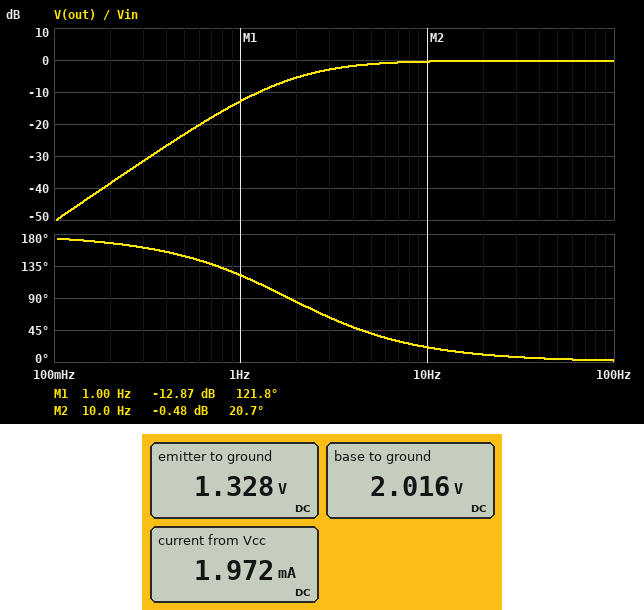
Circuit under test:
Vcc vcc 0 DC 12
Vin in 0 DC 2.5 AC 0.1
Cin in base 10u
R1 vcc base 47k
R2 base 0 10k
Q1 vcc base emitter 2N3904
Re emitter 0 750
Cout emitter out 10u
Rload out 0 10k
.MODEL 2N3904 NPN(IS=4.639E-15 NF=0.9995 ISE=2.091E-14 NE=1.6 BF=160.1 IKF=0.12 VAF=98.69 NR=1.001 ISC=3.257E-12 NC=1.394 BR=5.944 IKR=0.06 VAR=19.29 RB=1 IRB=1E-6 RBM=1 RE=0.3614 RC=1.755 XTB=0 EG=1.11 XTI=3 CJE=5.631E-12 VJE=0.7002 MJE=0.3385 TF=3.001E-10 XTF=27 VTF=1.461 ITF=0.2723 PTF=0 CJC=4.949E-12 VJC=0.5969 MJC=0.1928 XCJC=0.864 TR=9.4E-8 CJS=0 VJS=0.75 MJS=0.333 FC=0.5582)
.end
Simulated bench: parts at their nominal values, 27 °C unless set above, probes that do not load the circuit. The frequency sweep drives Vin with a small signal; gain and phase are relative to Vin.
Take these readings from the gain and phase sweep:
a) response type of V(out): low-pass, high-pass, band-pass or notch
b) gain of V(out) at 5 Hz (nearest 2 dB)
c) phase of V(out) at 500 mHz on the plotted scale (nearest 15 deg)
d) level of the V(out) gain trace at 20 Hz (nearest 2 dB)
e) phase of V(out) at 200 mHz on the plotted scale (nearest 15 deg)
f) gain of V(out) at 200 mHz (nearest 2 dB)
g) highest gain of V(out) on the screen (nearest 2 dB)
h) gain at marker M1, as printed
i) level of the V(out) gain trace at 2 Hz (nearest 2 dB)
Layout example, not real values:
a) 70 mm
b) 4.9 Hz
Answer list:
a) high-pass
b) -2 dB
c) 150 deg
d) 0 dB
e) 165 deg
f) -38 dB
g) 0 dB
h) -12.87 dB
i) -6 dB
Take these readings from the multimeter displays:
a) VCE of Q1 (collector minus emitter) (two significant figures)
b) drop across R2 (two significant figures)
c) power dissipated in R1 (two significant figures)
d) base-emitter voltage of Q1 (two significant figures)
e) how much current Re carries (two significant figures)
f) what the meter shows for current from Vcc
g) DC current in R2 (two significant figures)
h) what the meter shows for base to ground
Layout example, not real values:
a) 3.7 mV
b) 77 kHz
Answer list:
a) 11 V
b) 2.0 V
c) 2.1 mW
d) 690 mV
e) 1.8 mA
f) 1.972 mA
g) 200 µA
h) 2.016 V
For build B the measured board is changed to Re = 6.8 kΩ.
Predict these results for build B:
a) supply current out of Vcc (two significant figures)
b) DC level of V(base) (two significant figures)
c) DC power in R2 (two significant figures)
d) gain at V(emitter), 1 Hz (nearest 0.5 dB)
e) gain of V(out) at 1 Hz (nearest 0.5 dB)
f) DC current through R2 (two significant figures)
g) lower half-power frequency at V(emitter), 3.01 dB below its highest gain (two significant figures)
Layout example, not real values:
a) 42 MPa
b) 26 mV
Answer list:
a) 420 µA
b) 2.1 V
c) 440 µW
d) -7.0 dB
e) -12.5 dB
f) 210 µA
g) 1.9 Hz
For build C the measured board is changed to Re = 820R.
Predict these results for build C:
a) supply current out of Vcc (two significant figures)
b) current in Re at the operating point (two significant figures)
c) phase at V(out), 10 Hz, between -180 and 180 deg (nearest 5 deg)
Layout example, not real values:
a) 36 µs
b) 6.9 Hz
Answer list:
a) 1.8 mA
b) 1.6 mA
c) 20 deg
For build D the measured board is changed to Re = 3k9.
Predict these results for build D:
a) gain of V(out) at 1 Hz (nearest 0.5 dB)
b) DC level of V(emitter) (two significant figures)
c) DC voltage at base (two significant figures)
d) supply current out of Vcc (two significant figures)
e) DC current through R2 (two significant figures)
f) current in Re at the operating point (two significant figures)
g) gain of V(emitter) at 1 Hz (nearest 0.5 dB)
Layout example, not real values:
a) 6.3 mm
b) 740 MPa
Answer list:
a) -12.5 dB
b) 1.4 V
c) 2.1 V
d) 580 µA
e) 210 µA
f) 370 µA
g) -7.0 dB
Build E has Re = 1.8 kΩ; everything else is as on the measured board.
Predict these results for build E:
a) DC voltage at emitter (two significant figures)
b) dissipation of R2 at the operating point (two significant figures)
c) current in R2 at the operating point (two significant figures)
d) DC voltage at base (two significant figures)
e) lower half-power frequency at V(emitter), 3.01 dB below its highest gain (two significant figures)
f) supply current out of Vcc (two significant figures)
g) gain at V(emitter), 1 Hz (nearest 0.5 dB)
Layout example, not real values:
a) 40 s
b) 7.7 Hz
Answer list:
a) 1.4 V
b) 430 µW
c) 210 µA
d) 2.1 V
e) 2.0 Hz
f) 980 µA
g) -7.0 dB
